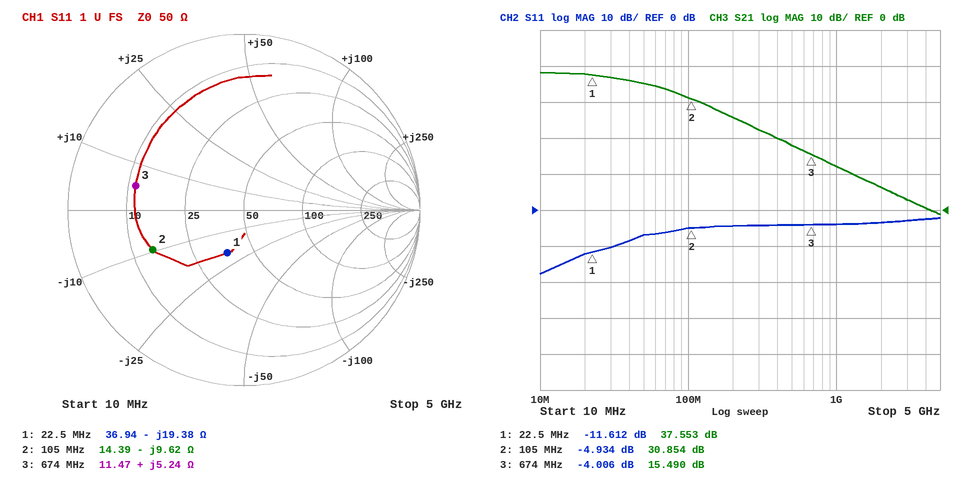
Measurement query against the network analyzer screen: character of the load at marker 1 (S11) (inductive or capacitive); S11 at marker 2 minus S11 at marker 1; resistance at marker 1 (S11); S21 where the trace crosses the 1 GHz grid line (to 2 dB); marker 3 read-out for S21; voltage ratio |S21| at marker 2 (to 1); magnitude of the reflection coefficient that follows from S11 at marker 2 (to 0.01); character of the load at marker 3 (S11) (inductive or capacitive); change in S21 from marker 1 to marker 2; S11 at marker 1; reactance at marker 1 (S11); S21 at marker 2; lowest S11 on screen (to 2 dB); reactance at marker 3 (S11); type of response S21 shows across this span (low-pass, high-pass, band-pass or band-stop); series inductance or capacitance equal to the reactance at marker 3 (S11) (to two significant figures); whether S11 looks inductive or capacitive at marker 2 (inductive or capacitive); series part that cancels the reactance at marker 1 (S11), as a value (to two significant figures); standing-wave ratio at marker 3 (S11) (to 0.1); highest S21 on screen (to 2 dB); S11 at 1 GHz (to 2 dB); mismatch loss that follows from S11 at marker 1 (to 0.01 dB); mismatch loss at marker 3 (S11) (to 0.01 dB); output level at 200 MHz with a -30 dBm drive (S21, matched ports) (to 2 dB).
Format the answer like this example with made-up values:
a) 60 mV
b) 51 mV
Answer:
a) capacitive
b) 6.678 dB
c) 36.94 Ω
d) 12 dB
e) 15.490 dB
f) 35
g) 0.57
h) inductive
i) -6.699 dB
j) -11.612 dB
k) -19.38 Ω
l) 30.854 dB
m) -18 dB
n) +5.24 Ω
o) low-pass
p) 1.2 nH
q) capacitive
r) 140 nH
s) 4.4
t) 38 dB
u) -4 dB
v) 0.31 dB
w) 2.20 dB
x) -4 dBm
